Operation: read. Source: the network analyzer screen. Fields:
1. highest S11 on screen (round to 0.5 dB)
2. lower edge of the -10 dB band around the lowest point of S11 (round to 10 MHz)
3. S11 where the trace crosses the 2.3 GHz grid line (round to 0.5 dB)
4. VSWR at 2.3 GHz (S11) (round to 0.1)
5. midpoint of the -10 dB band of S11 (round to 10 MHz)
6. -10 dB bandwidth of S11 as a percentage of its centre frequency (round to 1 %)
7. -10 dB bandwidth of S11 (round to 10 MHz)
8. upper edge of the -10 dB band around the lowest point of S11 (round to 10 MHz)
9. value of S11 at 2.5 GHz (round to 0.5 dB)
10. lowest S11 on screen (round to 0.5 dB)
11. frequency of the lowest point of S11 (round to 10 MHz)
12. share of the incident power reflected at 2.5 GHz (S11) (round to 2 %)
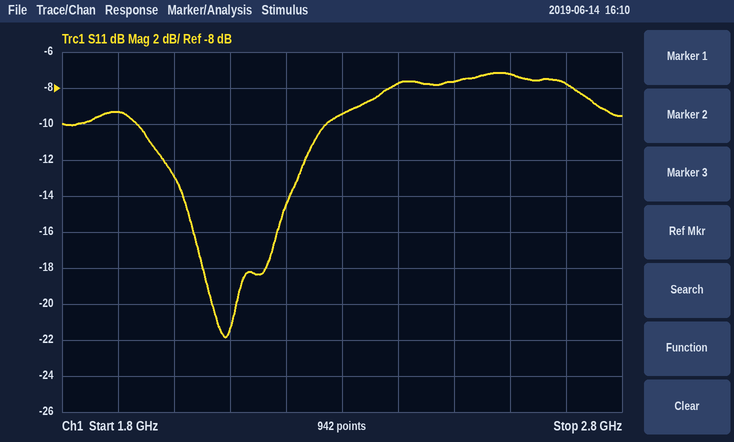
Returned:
-7.0 dB
1.93 GHz
-9.5 dB
2.0
2.10 GHz
16 %
340 MHz
2.27 GHz
-7.5 dB
-22.0 dB
2.09 GHz
18 %
